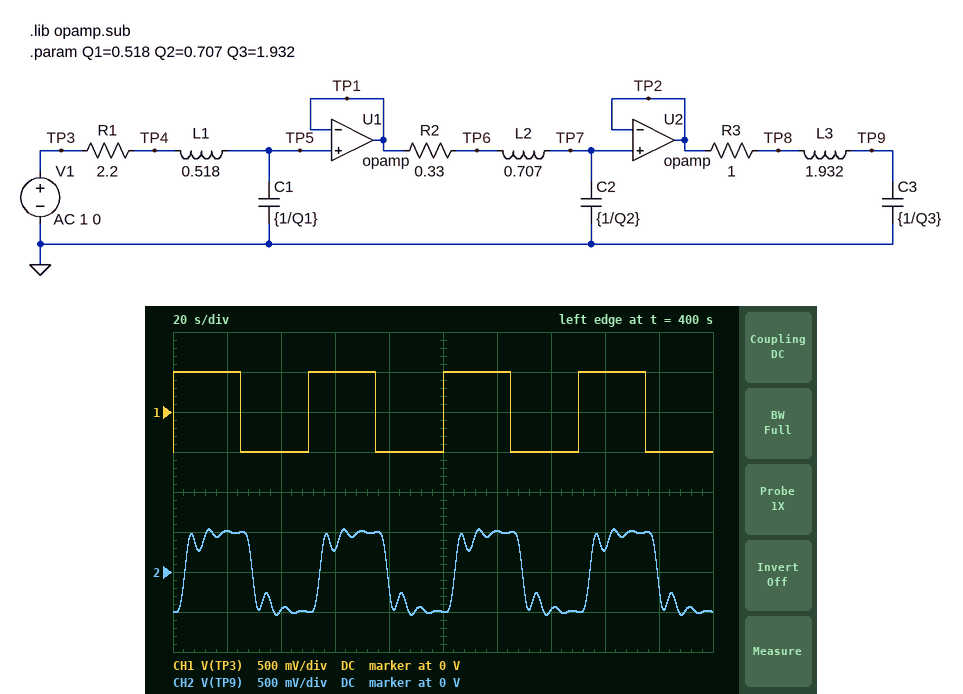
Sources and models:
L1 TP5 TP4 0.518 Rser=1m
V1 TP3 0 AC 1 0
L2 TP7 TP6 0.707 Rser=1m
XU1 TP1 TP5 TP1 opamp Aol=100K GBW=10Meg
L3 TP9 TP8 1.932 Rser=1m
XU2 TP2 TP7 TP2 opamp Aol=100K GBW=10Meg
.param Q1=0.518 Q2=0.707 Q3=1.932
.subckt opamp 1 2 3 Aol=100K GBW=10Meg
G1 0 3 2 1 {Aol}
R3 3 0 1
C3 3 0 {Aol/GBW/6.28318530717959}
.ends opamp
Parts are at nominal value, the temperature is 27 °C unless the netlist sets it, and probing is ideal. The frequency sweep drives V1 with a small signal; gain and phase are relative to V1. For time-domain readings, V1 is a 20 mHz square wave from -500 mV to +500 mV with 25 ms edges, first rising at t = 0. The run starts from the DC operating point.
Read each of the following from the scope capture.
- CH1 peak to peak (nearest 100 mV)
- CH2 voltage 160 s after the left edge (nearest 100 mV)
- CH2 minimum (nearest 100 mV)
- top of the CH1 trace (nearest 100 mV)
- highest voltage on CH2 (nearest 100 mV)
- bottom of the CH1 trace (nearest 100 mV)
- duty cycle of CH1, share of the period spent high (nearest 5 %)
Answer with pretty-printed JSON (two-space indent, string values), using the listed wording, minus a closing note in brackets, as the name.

{
  "CH1 peak to peak": "1.0 V",
  "CH2 voltage 160 s after the left edge": "300 mV",
  "CH2 minimum": "-500 mV",
  "top of the CH1 trace": "500 mV",
  "highest voltage on CH2": "500 mV",
  "bottom of the CH1 trace": "-500 mV",
  "duty cycle of CH1, share of the period spent high": "50 %"
}
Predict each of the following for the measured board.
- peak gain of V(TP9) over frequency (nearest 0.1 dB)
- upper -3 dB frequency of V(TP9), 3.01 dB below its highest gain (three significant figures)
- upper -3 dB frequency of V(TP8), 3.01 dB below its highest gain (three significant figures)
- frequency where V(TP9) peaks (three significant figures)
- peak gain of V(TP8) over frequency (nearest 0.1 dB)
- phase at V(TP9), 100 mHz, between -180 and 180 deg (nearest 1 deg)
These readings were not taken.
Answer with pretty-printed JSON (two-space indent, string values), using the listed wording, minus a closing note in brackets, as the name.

{
  "peak gain of V(TP9) over frequency": "1.0 dB",
  "upper -3 dB frequency of V(TP9), 3.01 dB below its highest gain": "168 mHz",
  "upper -3 dB frequency of V(TP8), 3.01 dB below its highest gain": "44.3 mHz",
  "frequency where V(TP9) peaks": "143 mHz",
  "peak gain of V(TP8) over frequency": "0 dB",
  "phase at V(TP9), 100 mHz, between -180 and 180 deg": "-131 deg"
}
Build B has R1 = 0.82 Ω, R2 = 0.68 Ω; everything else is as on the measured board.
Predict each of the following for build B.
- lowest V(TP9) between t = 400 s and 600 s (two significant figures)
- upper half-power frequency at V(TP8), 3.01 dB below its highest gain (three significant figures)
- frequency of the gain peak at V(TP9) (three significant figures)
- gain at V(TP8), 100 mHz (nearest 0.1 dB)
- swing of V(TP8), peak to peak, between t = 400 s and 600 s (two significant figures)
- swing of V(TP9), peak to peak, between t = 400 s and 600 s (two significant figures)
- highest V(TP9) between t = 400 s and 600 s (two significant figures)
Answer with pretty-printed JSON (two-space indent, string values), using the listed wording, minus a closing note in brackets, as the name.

{
  "lowest V(TP9) between t = 400 s and 600 s": "-880 mV",
  "upper half-power frequency at V(TP8), 3.01 dB below its highest gain": "118 mHz",
  "frequency of the gain peak at V(TP9)": "130 mHz",
  "gain at V(TP8), 100 mHz": "-1.1 dB",
  "swing of V(TP8), peak to peak, between t = 400 s and 600 s": "1.3 V",
  "swing of V(TP9), peak to peak, between t = 400 s and 600 s": "1.8 V",
  "highest V(TP9) between t = 400 s and 600 s": "880 mV"
}
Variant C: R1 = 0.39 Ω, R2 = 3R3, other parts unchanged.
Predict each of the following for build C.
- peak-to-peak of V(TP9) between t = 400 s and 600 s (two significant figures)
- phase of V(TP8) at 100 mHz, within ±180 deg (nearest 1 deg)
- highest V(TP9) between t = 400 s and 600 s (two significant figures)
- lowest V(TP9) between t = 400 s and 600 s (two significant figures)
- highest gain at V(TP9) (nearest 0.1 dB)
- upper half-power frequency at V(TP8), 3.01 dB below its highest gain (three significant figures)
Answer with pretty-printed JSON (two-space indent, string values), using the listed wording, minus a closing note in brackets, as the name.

{
  "peak-to-peak of V(TP9) between t = 400 s and 600 s": "990 mV",
  "phase of V(TP8) at 100 mHz, within ±180 deg": "-145 deg",
  "highest V(TP9) between t = 400 s and 600 s": "500 mV",
  "lowest V(TP9) between t = 400 s and 600 s": "-500 mV",
  "highest gain at V(TP9)": "0 dB",
  "upper half-power frequency at V(TP8), 3.01 dB below its highest gain": "38.0 mHz"
}
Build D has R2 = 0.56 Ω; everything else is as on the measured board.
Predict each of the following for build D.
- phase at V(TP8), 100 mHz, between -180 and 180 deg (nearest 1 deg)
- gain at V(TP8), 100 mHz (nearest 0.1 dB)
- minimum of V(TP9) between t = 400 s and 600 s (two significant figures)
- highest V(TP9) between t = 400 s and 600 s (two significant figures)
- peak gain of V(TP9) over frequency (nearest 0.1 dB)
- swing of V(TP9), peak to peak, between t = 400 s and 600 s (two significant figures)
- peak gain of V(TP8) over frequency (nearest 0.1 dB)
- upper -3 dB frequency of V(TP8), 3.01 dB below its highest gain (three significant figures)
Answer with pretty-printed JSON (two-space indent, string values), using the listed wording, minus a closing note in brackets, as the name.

{
  "phase at V(TP8), 100 mHz, between -180 and 180 deg": "-145 deg",
  "gain at V(TP8), 100 mHz": "-7.7 dB",
  "minimum of V(TP9) between t = 400 s and 600 s": "-500 mV",
  "highest V(TP9) between t = 400 s and 600 s": "500 mV",
  "peak gain of V(TP9) over frequency": "0 dB",
  "swing of V(TP9), peak to peak, between t = 400 s and 600 s": "1.0 V",
  "peak gain of V(TP8) over frequency": "0 dB",
  "upper -3 dB frequency of V(TP8), 3.01 dB below its highest gain": "42.6 mHz"
}
